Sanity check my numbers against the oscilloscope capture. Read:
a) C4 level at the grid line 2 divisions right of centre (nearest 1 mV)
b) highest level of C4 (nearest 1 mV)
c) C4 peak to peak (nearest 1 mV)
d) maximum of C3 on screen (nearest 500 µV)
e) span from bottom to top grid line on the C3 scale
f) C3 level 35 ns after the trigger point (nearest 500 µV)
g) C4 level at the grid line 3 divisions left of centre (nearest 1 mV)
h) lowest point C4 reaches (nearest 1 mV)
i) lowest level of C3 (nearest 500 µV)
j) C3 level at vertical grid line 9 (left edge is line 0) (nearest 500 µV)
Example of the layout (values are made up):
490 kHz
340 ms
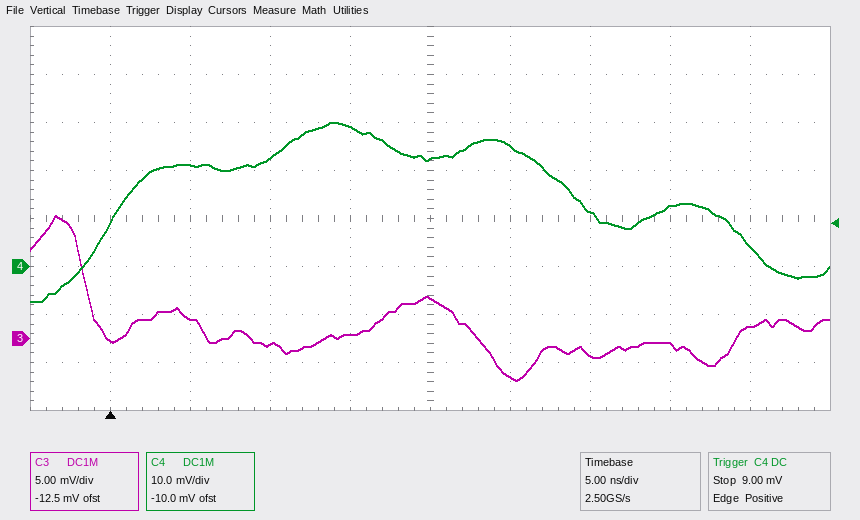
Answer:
11 mV
30 mV
37 mV
13.0 mV
40 mV
-500 µV
21 mV
-7 mV
-4.5 mV
1.0 mV
